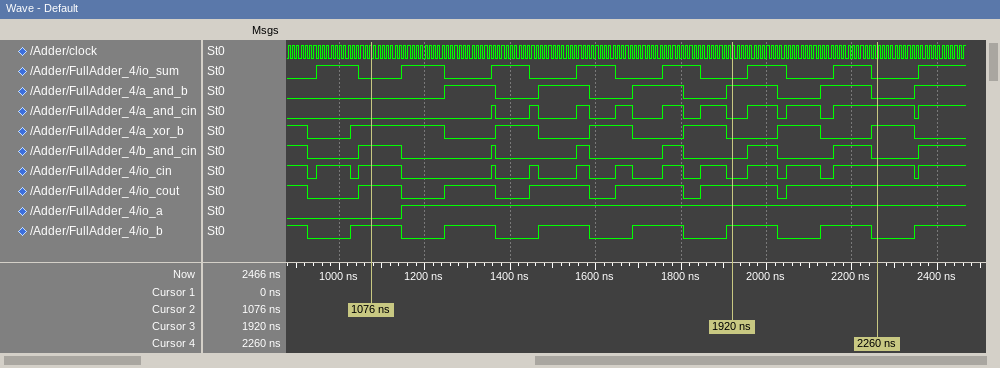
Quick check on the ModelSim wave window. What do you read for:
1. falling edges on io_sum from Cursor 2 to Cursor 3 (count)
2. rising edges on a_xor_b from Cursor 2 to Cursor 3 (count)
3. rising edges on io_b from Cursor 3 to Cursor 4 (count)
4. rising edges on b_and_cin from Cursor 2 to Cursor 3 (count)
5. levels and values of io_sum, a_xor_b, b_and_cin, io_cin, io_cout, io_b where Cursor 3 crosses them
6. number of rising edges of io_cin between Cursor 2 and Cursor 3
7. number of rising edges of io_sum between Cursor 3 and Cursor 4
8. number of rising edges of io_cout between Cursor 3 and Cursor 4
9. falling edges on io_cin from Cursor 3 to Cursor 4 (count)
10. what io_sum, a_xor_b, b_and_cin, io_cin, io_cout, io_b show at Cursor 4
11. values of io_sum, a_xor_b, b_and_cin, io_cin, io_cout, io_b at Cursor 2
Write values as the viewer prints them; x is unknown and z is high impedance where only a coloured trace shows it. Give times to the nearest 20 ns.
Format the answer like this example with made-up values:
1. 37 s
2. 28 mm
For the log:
1. 4
2. 3
3. 1
4. 3
5. io_sum=0, a_xor_b=0, b_and_cin=0, io_cin=0, io_cout=1, io_b=1
6. 6
7. 2
8. 1
9. 2
10. io_sum=0, a_xor_b=1, b_and_cin=0, io_cin=1, io_cout=1, io_b=0
11. io_sum=0, a_xor_b=1, b_and_cin=1, io_cin=1, io_cout=1, io_b=1
